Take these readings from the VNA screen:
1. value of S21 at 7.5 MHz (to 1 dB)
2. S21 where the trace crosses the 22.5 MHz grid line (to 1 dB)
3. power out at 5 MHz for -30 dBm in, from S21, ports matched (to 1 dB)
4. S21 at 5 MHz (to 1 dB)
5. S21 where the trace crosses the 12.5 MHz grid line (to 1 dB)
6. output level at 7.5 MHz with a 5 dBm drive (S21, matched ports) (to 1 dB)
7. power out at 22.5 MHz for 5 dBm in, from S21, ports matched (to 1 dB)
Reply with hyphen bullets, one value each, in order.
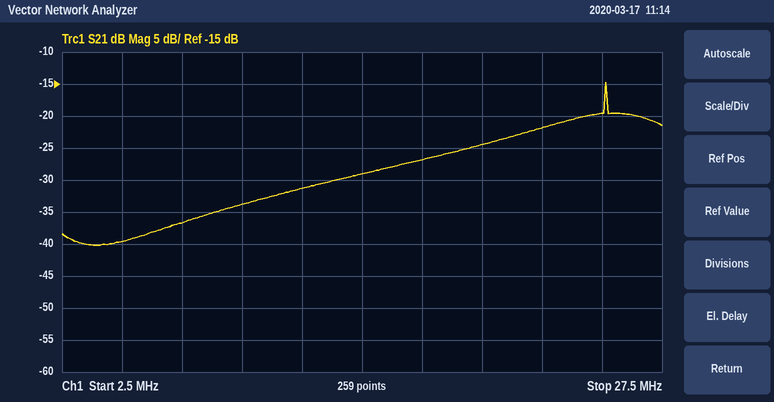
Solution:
- -37 dB
- -22 dB
- -70 dBm
- -40 dB
- -31 dB
- -32 dBm
- -17 dBm
